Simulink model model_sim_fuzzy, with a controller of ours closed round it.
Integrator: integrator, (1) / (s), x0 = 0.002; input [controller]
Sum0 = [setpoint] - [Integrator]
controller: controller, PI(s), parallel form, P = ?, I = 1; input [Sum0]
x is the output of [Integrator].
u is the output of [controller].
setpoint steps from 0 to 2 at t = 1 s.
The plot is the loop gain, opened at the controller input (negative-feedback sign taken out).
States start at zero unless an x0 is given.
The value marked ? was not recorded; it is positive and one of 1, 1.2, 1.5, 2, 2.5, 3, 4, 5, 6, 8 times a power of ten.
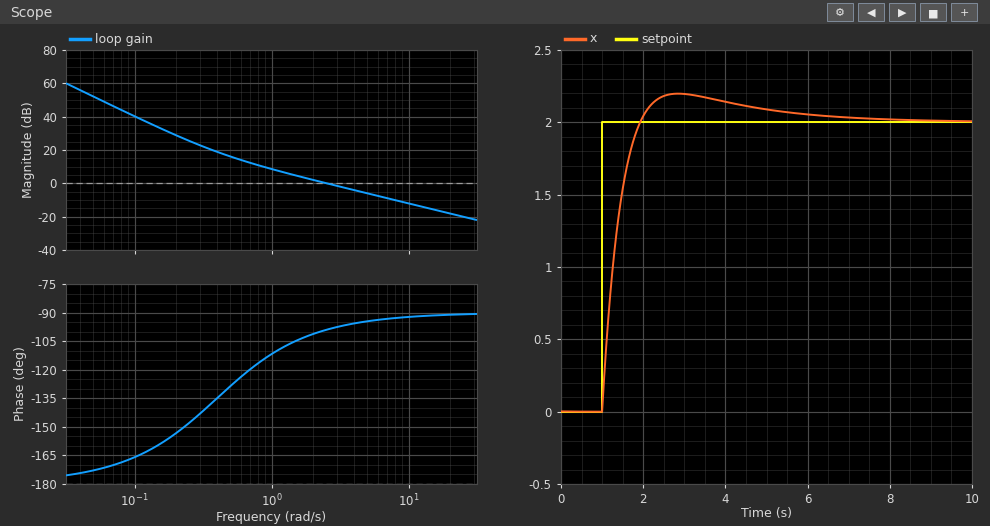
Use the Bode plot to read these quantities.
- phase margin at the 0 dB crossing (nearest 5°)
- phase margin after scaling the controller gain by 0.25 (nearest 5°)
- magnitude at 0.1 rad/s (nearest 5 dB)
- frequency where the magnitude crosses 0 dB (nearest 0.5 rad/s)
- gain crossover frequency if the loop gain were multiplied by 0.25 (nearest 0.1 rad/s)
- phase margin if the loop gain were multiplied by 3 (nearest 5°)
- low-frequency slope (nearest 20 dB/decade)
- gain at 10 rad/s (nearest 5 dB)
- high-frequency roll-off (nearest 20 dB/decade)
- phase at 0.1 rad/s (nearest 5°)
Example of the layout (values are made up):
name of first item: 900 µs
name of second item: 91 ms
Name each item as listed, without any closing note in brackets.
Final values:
phase margin at the 0 dB crossing: 80°
phase margin after scaling the controller gain by 0.25: 60°
magnitude at 0.1 rad/s: 40 dB
frequency where the magnitude crosses 0 dB: 2.5 rad/s
gain crossover frequency if the loop gain were multiplied by 0.25: 0.7 rad/s
phase margin if the loop gain were multiplied by 3: 85°
low-frequency slope: -40 dB/decade
gain at 10 rad/s: -10 dB
high-frequency roll-off: -20 dB/decade
phase at 0.1 rad/s: -165°
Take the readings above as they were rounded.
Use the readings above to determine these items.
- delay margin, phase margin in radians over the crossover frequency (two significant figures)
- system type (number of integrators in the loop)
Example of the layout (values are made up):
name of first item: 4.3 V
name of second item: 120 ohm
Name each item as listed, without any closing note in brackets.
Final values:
delay margin, phase margin in radians over the crossover frequency: 0.56 s
system type: 2
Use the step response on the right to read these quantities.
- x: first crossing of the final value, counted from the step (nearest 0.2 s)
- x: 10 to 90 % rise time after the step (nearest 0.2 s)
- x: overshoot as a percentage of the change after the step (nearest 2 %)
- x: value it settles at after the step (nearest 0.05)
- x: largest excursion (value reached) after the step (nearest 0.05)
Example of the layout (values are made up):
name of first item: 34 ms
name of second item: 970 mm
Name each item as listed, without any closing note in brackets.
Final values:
x: first crossing of the final value, counted from the step: 1.0 s
x: 10 to 90 % rise time after the step: 0.6 s
x: overshoot as a percentage of the change after the step: 10 %
x: value it settles at after the step: 2.00
x: largest excursion (value reached) after the step: 2.20
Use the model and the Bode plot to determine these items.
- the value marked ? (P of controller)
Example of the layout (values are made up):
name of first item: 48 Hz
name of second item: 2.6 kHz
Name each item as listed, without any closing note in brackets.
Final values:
the value marked ?: 2.5
